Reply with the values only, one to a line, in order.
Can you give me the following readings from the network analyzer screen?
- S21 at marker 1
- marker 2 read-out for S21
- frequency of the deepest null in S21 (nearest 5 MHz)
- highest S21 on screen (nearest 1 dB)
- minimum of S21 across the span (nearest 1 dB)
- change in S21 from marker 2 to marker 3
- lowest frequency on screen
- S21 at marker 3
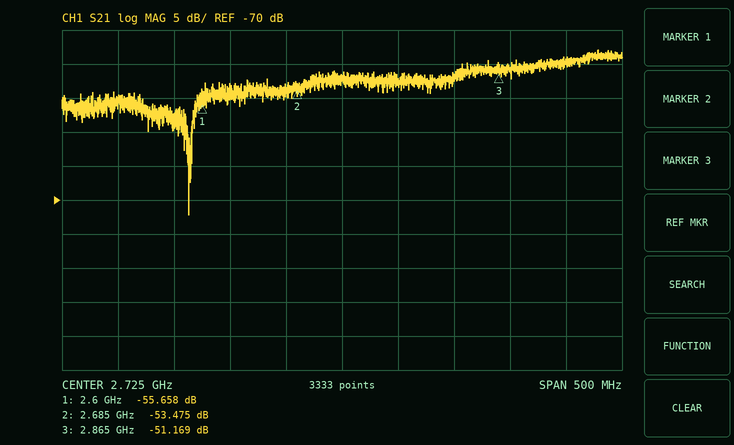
-55.658 dB
-53.475 dB
2.590 GHz
-48 dB
-72 dB
2.306 dB
2.475 GHz
-51.169 dB
